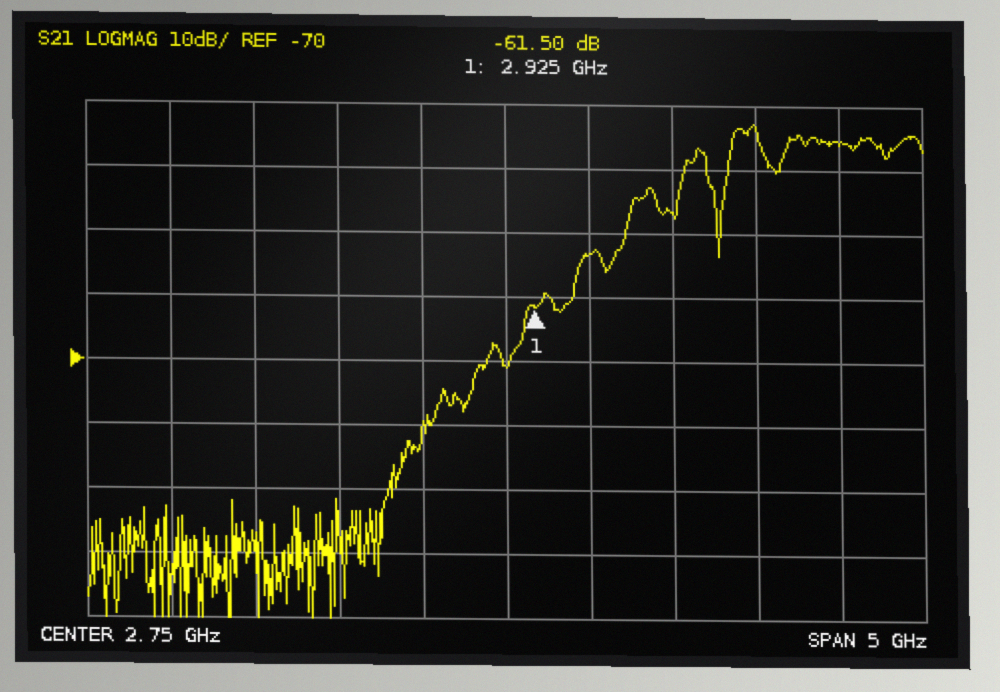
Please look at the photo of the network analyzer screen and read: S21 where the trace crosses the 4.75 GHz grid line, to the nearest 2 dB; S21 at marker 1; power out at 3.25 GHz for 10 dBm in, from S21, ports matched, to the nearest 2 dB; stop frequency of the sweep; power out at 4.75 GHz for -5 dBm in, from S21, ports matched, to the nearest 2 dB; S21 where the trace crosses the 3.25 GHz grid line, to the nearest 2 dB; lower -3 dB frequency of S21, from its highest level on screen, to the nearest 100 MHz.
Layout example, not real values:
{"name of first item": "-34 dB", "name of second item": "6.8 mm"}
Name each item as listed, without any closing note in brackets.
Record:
{"S21 where the trace crosses the 4.75 GHz grid line, to the nearest 2 dB": "-36 dB", "S21 at marker 1": "-61.50 dB", "power out at 3.25 GHz for 10 dBm in, from S21, ports matched, to the nearest 2 dB": "-44 dBm", "stop frequency of the sweep": "5.25 GHz", "power out at 4.75 GHz for -5 dBm in, from S21, ports matched, to the nearest 2 dB": "-40 dBm", "S21 where the trace crosses the 3.25 GHz grid line, to the nearest 2 dB": "-54 dB", "lower -3 dB frequency of S21, from its highest level on screen, to the nearest 100 MHz": "4.1 GHz"}
